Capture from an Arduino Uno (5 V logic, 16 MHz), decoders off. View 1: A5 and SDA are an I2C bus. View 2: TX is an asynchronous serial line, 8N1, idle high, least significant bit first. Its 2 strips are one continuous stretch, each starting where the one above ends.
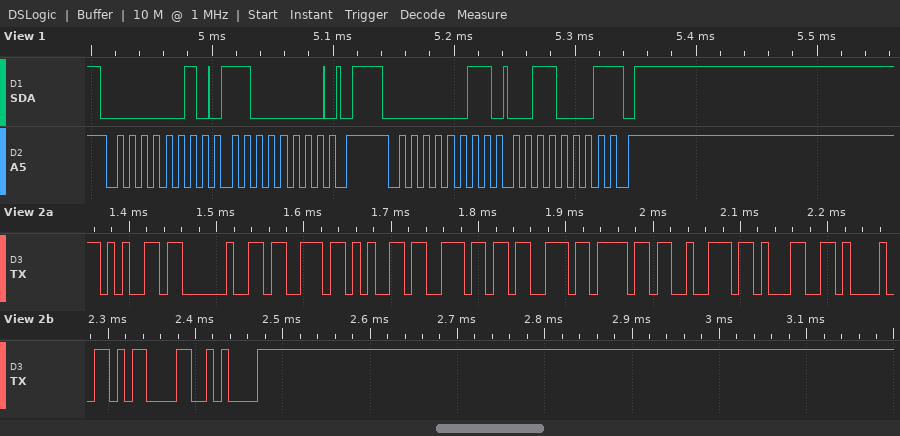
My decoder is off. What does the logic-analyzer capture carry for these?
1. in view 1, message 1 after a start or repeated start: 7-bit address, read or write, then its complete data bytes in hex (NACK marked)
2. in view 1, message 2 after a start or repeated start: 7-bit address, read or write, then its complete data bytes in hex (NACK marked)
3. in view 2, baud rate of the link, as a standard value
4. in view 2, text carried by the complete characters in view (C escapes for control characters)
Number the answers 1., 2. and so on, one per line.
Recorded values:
1. 0x01 write: C0
2. 0x01 read: 31 NACK
3. 115200 baud
4. "e sensor1!\r\n"
